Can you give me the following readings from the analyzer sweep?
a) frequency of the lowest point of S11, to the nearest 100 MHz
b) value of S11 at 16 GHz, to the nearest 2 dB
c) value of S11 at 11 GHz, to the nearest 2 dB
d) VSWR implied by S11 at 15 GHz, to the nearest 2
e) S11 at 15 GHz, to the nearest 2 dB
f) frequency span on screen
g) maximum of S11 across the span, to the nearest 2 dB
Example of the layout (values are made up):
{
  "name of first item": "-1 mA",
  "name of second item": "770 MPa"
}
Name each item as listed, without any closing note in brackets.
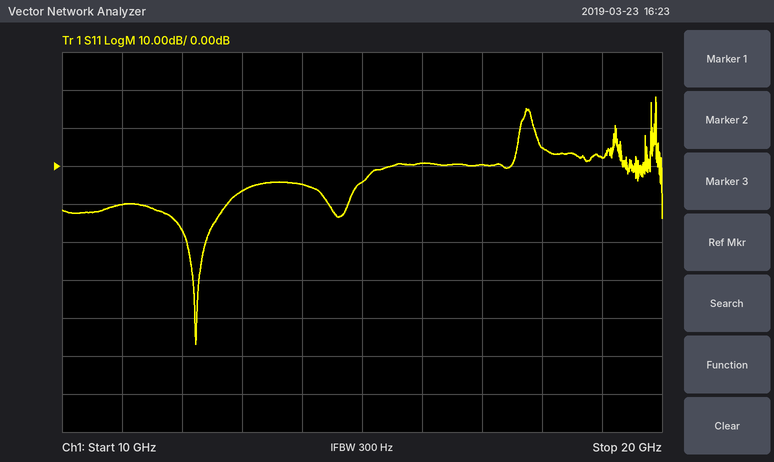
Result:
{
  "frequency of the lowest point of S11, to the nearest 100 MHz": "12.2 GHz",
  "value of S11 at 16 GHz, to the nearest 2 dB": "0 dB",
  "value of S11 at 11 GHz, to the nearest 2 dB": "-10 dB",
  "VSWR implied by S11 at 15 GHz, to the nearest 2": "4",
  "S11 at 15 GHz, to the nearest 2 dB": "-4 dB",
  "frequency span on screen": "10 GHz",
  "maximum of S11 across the span, to the nearest 2 dB": "18 dB"
}
